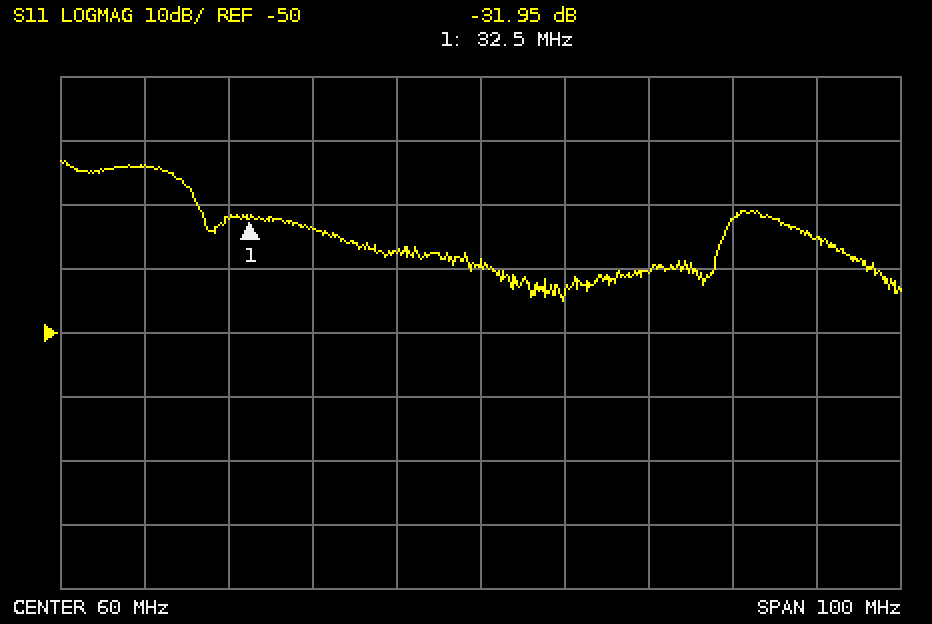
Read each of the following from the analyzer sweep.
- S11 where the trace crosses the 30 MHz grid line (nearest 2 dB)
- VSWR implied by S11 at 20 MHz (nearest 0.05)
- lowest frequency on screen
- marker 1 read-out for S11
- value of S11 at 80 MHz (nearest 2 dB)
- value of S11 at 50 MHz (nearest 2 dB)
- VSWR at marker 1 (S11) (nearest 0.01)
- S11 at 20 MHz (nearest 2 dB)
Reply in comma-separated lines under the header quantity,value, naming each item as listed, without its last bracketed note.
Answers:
quantity,value
S11 where the trace crosses the 30 MHz grid line,-32 dB
VSWR implied by S11 at 20 MHz,1.15
lowest frequency on screen,10 MHz
marker 1 read-out for S11,-31.95 dB
value of S11 at 80 MHz,-40 dB
value of S11 at 50 MHz,-38 dB
VSWR at marker 1 (S11),1.05
S11 at 20 MHz,-24 dB
